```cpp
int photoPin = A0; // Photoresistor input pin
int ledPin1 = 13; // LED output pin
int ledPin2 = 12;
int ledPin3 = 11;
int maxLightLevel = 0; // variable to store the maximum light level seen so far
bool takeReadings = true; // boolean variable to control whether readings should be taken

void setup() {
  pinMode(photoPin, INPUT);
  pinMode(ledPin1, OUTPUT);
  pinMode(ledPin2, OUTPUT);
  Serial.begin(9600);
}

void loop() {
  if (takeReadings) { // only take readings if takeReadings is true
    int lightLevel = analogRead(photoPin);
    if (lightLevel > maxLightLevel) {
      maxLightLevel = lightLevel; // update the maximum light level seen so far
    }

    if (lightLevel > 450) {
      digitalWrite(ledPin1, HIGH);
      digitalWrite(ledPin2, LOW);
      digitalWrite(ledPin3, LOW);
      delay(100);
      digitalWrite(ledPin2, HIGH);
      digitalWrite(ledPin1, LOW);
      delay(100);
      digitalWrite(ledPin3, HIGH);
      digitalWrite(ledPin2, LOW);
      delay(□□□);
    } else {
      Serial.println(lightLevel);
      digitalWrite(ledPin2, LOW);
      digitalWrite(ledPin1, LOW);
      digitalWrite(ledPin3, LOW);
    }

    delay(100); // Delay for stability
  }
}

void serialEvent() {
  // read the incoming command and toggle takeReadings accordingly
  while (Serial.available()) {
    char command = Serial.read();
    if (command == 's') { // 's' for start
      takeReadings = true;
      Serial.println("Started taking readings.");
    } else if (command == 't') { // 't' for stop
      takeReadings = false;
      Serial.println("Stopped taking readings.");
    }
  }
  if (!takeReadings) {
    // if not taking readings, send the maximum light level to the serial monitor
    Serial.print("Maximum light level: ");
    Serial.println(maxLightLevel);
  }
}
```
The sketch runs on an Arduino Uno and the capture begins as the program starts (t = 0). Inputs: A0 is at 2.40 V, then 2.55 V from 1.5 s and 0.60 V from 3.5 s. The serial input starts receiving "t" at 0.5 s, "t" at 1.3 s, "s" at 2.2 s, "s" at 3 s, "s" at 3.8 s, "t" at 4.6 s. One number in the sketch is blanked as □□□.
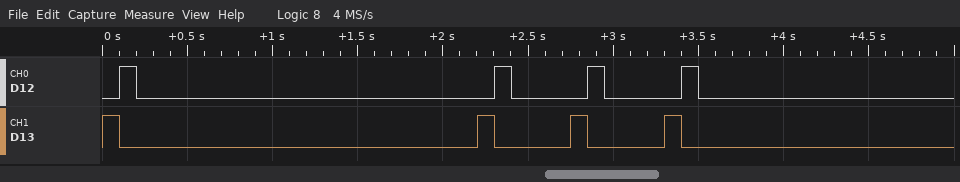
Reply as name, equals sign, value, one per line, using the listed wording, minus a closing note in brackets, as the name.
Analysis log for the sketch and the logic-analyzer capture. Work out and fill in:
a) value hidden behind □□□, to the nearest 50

value hidden behind □□□, to the nearest 50 = 250
